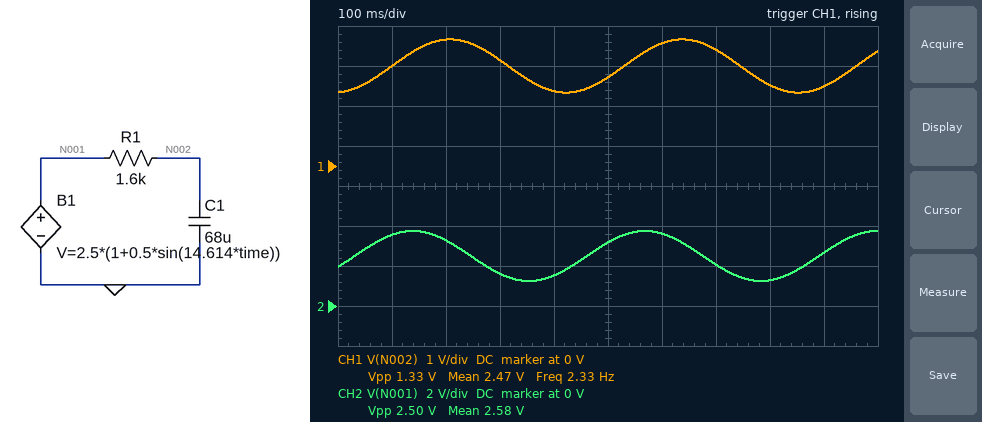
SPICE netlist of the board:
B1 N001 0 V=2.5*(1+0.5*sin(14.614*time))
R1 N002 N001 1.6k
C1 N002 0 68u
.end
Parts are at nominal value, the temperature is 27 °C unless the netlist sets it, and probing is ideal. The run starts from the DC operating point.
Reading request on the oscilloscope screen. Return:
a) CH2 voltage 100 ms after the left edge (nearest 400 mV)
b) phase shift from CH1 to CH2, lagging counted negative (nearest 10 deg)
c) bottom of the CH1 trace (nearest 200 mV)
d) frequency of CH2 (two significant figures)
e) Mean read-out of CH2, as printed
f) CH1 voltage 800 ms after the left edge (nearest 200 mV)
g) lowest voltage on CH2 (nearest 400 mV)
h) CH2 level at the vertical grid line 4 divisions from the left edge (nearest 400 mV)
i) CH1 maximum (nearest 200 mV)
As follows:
3.6 V
60 deg
1.8 V
2.3 Hz
2.58 V
2.0 V
1.2 V
1.6 V
3.2 V
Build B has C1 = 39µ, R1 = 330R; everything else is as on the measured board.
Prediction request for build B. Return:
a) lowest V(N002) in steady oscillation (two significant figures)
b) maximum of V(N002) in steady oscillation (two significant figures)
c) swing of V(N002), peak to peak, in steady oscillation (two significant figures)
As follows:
1.3 V
3.7 V
2.5 V
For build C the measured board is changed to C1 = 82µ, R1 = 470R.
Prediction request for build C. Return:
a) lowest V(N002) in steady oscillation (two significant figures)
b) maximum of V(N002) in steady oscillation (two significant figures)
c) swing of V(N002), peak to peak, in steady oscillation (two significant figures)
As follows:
1.4 V
3.6 V
2.2 V
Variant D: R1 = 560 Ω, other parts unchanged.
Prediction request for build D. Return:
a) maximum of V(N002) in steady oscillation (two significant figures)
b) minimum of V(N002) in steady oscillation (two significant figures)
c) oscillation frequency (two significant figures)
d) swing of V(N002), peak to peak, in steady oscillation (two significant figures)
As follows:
3.6 V
1.4 V
2.3 Hz
2.2 V
